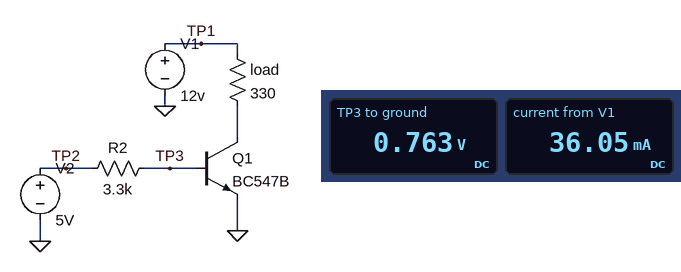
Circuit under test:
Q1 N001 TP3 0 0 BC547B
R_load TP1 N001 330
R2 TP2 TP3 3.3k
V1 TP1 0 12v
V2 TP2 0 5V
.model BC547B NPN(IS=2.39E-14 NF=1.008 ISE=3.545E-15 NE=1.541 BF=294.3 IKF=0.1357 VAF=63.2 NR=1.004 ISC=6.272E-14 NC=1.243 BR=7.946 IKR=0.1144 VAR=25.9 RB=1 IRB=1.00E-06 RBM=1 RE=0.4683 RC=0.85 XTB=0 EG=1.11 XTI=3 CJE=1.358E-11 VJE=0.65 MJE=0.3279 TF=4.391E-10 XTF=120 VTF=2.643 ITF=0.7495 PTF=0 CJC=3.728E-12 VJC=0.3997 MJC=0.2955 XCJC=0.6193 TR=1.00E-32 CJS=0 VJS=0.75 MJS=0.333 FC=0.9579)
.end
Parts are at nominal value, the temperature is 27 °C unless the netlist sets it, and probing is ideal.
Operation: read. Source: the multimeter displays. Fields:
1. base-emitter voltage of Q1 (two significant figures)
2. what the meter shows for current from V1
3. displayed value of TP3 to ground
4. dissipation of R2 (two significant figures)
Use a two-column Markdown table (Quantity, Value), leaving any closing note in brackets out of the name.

| Quantity | Value |
|---|---|
| base-emitter voltage of Q1 | 760 mV |
| what the meter shows for current from V1 | 36.05 mA |
| displayed value of TP3 to ground | 0.763 V |
| dissipation of R2 | 5.4 mW |
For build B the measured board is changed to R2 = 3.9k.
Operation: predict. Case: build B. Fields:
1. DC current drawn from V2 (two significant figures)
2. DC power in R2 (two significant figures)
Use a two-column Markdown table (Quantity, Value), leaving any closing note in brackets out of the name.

| Quantity | Value |
|---|---|
| DC current drawn from V2 | 1.1 mA |
| DC power in R2 | 4.6 mW |
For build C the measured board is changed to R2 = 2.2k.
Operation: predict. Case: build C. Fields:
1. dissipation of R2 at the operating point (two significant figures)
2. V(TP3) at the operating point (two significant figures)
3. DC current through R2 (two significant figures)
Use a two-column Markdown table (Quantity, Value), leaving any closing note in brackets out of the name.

| Quantity | Value |
|---|---|
| dissipation of R2 at the operating point | 8.1 mW |
| V(TP3) at the operating point | 770 mV |
| DC current through R2 | 1.9 mA |
